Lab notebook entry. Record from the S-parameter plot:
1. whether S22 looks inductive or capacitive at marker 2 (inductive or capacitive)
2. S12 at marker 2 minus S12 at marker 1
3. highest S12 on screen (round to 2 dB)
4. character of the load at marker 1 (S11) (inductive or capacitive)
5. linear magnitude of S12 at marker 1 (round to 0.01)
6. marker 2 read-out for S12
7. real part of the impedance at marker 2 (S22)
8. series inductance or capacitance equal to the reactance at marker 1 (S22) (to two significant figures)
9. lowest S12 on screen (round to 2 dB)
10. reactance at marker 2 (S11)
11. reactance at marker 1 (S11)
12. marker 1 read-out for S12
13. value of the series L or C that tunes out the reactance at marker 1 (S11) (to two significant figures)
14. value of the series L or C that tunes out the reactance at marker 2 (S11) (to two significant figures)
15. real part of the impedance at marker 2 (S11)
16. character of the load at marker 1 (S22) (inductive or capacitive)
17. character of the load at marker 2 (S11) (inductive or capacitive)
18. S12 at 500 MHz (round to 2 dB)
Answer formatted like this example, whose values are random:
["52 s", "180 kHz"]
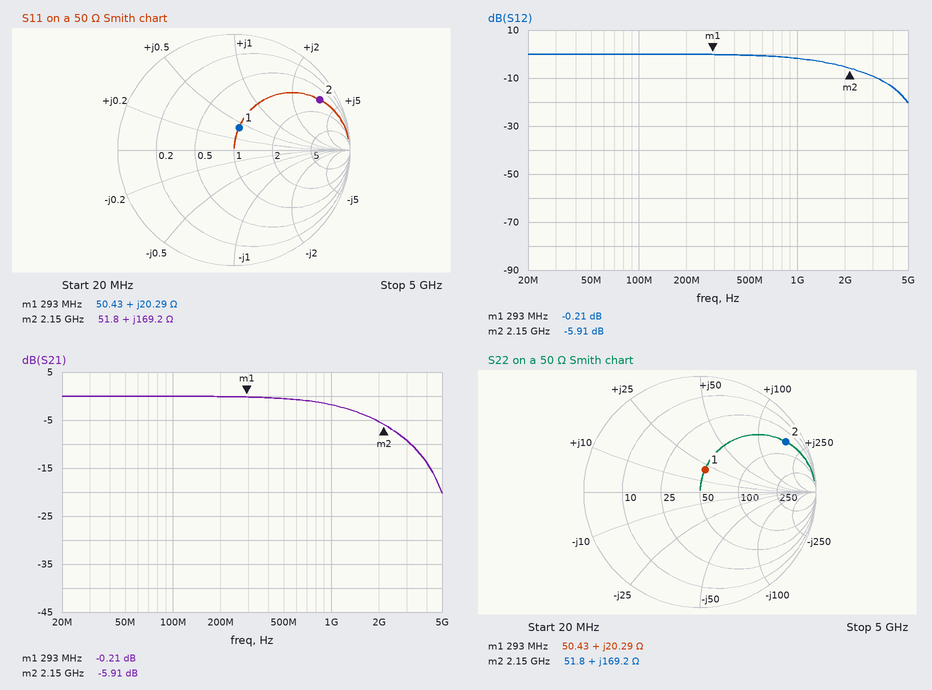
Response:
["inductive", "-5.70 dB", "0 dB", "inductive", "0.98", "-5.91 dB", "51.8 Ω", "11 nH", "-20 dB", "+169.2 Ω", "+20.29 Ω", "-0.21 dB", "27 pF", "440 fF", "51.8 Ω", "inductive", "inductive", "0 dB"]
